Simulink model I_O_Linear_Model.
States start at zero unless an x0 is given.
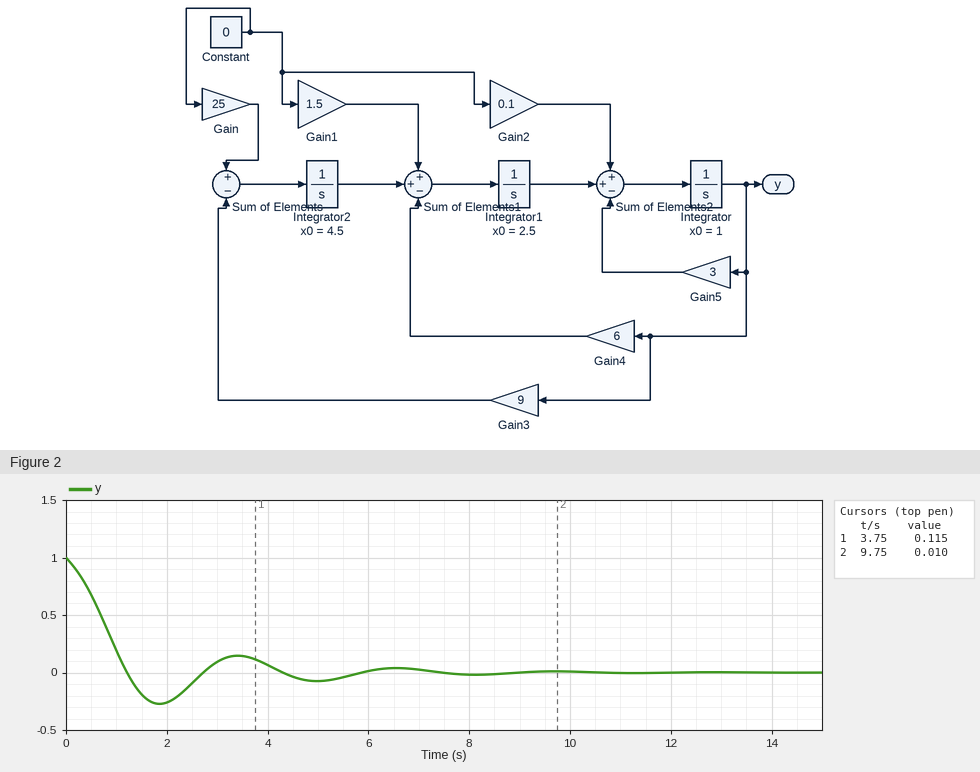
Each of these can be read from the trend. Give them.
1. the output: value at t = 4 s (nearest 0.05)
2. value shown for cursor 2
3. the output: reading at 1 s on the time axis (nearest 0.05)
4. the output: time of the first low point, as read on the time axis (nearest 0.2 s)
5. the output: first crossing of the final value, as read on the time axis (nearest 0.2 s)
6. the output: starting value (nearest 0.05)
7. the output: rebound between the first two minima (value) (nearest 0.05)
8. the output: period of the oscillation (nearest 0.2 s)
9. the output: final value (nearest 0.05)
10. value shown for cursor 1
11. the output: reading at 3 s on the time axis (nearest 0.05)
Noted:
0.05
0.010
0.20
1.8 s
1.2 s
1.00
0.15
3.2 s
0.00
0.115
0.10
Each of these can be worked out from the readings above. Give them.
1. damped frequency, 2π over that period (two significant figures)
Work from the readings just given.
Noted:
2.0 rad/s
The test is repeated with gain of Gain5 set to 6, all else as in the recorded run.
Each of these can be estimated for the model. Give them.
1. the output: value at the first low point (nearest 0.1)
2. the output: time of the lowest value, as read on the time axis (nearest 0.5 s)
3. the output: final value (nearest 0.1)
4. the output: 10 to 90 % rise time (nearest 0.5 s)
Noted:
-0.1
3.0 s
0.0
1.5 s
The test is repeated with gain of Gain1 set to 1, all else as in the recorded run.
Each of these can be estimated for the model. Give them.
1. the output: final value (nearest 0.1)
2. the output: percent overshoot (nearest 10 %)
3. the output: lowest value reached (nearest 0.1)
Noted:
0.0
30 %
-0.3
